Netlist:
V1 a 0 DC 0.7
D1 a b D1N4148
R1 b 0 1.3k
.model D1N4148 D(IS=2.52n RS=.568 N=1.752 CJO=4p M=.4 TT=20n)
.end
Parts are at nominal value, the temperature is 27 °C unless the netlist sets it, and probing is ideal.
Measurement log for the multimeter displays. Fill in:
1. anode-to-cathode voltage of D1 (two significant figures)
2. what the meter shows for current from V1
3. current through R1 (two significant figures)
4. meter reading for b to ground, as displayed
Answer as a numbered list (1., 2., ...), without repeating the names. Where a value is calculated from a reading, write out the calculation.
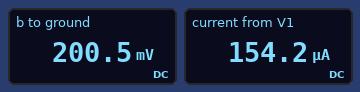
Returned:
1. 700 mV - 200.5 mV = 500 mV
2. 154.2 µA
3. (200.5 mV) / 1.3 kΩ = 150 µA
4. 200.5 mV
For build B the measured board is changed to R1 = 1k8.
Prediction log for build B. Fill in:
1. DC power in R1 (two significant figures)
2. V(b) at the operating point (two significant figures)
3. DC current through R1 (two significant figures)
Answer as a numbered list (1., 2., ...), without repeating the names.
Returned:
1. 25 µW
2. 210 mV
3. 120 µA
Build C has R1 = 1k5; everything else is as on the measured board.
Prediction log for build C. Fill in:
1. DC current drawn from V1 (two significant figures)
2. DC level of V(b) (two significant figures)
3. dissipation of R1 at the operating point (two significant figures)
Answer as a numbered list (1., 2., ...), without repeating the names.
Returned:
1. 140 µA
2. 210 mV
3. 28 µW
